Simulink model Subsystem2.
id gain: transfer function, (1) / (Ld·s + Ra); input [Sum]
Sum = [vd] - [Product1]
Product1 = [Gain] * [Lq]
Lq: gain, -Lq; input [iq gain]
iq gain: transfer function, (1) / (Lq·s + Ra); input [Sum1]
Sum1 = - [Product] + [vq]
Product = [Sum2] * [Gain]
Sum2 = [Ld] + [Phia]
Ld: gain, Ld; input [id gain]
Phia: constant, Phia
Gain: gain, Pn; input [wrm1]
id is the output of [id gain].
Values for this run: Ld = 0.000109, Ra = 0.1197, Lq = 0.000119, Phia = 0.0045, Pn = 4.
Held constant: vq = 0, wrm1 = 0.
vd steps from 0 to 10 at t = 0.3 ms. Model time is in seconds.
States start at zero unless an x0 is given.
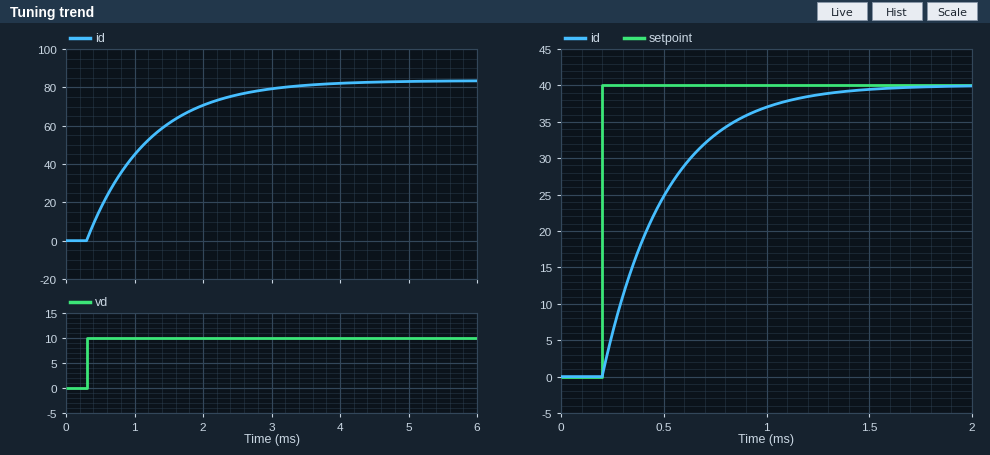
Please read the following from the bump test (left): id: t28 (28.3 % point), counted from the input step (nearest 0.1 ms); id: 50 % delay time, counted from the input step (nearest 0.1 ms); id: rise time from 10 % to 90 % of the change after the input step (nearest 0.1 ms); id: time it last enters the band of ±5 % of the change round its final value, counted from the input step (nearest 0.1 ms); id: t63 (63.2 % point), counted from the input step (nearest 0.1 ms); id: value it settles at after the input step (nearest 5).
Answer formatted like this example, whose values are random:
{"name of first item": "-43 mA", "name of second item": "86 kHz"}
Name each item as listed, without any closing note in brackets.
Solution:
{"id: t28 (28.3 % point), counted from the input step": "0.3 ms", "id: 50 % delay time, counted from the input step": "0.6 ms", "id: rise time from 10 % to 90 % of the change after the input step": "2.0 ms", "id: time it last enters the band of ±5 % of the change round its final value, counted from the input step": "2.7 ms", "id: t63 (63.2 % point), counted from the input step": "0.9 ms", "id: value it settles at after the input step": "85"}
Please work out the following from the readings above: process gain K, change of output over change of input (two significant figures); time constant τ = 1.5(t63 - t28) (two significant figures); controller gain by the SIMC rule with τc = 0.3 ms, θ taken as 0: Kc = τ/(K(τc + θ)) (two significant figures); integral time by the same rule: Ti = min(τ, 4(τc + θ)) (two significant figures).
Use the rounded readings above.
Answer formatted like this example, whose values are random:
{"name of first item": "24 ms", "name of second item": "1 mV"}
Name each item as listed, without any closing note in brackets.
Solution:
{"process gain K, change of output over change of input": "8.5", "time constant τ = 1.5(t63 - t28)": "0.90 ms", "controller gain by the SIMC rule with τc = 0.3 ms, θ taken as 0: Kc = τ/(K(τc + θ))": "0.35", "integral time by the same rule: Ti = min(τ, 4(τc + θ))": "0.90 ms"}
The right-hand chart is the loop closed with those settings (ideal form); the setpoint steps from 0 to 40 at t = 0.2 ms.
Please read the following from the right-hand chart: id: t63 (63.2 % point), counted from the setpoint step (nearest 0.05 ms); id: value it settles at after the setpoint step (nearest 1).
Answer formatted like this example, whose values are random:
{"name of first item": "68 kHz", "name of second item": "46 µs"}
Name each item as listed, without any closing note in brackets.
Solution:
{"id: t63 (63.2 % point), counted from the setpoint step": "0.30 ms", "id: value it settles at after the setpoint step": "40"}
